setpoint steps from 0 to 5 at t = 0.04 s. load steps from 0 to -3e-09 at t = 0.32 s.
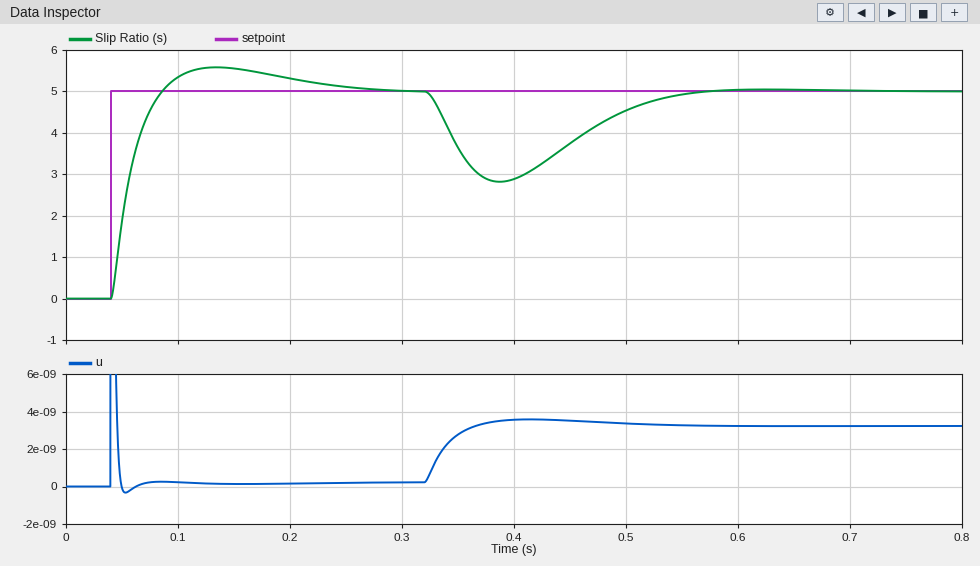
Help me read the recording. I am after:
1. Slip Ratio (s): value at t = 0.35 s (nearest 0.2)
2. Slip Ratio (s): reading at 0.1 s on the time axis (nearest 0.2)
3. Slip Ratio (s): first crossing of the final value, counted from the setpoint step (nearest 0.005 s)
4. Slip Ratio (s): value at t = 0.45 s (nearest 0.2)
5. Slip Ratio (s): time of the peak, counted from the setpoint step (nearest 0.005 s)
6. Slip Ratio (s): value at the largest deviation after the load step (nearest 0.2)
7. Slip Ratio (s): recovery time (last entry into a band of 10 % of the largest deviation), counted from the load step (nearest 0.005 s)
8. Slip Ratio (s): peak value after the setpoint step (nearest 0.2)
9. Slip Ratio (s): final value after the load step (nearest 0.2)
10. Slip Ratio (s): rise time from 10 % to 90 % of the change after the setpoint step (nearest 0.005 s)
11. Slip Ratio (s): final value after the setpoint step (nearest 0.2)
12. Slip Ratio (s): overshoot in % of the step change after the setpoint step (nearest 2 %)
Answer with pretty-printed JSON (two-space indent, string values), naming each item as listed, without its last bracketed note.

{
  "Slip Ratio (s): value at t = 0.35 s": "3.6",
  "Slip Ratio (s): reading at 0.1 s on the time axis": "5.4",
  "Slip Ratio (s): first crossing of the final value, counted from the setpoint step": "0.045 s",
  "Slip Ratio (s): value at t = 0.45 s": "3.8",
  "Slip Ratio (s): time of the peak, counted from the setpoint step": "0.095 s",
  "Slip Ratio (s): value at the largest deviation after the load step": "2.8",
  "Slip Ratio (s): recovery time (last entry into a band of 10 % of the largest deviation), counted from the load step": "0.205 s",
  "Slip Ratio (s): peak value after the setpoint step": "5.6",
  "Slip Ratio (s): final value after the load step": "5.0",
  "Slip Ratio (s): rise time from 10 % to 90 % of the change after the setpoint step": "0.030 s",
  "Slip Ratio (s): final value after the setpoint step": "5.0",
  "Slip Ratio (s): overshoot in % of the step change after the setpoint step": "12 %"
}
